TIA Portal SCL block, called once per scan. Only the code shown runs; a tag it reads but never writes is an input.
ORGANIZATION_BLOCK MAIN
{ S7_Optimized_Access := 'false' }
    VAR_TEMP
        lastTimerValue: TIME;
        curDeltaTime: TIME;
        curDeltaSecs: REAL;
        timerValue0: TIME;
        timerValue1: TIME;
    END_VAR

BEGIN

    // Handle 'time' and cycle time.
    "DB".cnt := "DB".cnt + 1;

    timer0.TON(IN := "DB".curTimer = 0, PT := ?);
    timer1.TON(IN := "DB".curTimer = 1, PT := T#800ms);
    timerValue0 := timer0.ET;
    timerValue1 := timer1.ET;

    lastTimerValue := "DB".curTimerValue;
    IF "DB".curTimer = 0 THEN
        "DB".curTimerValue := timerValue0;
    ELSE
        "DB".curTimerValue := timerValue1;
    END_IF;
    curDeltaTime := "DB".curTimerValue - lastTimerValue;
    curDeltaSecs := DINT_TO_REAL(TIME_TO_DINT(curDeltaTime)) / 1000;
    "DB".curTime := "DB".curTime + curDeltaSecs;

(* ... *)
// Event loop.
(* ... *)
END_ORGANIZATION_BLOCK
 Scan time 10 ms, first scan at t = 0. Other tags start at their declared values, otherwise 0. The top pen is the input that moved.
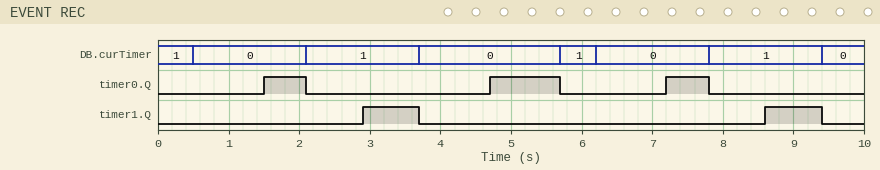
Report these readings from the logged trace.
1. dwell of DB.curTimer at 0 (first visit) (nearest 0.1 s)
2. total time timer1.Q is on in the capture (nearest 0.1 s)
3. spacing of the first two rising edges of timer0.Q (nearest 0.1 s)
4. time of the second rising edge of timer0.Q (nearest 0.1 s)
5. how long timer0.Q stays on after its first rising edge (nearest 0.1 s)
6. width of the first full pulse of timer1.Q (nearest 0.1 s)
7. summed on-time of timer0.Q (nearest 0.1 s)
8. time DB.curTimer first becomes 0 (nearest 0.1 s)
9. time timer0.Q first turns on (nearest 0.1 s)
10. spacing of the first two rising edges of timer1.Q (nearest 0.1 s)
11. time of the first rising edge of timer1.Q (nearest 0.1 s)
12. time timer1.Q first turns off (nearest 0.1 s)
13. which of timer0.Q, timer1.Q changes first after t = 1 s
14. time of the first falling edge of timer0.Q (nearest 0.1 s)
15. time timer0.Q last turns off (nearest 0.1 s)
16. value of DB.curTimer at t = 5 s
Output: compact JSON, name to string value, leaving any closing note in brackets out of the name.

{"dwell of DB.curTimer at 0 (first visit)": "1.6 s", "total time timer1.Q is on in the capture": "1.6 s", "spacing of the first two rising edges of timer0.Q": "3.2 s", "time of the second rising edge of timer0.Q": "4.7 s", "how long timer0.Q stays on after its first rising edge": "0.6 s", "width of the first full pulse of timer1.Q": "0.8 s", "summed on-time of timer0.Q": "2.2 s", "time DB.curTimer first becomes 0": "0.5 s", "time timer0.Q first turns on": "1.5 s", "spacing of the first two rising edges of timer1.Q": "5.7 s", "time of the first rising edge of timer1.Q": "2.9 s", "time timer1.Q first turns off": "3.7 s", "which of timer0.Q, timer1.Q changes first after t = 1 s": "timer0.Q", "time of the first falling edge of timer0.Q": "2.1 s", "time timer0.Q last turns off": "7.8 s", "value of DB.curTimer at t = 5 s": "0"}
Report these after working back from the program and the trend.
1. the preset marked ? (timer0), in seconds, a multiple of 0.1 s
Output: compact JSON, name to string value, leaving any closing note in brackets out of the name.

{"the preset marked ? (timer0), in seconds, a multiple of 0.1 s": "1.0 s"}
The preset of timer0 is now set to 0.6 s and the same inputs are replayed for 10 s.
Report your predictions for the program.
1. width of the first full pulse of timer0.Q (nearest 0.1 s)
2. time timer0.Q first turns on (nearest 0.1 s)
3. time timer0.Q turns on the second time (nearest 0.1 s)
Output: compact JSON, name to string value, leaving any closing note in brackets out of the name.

{"width of the first full pulse of timer0.Q": "1.0 s", "time timer0.Q first turns on": "1.1 s", "time timer0.Q turns on the second time": "4.3 s"}
